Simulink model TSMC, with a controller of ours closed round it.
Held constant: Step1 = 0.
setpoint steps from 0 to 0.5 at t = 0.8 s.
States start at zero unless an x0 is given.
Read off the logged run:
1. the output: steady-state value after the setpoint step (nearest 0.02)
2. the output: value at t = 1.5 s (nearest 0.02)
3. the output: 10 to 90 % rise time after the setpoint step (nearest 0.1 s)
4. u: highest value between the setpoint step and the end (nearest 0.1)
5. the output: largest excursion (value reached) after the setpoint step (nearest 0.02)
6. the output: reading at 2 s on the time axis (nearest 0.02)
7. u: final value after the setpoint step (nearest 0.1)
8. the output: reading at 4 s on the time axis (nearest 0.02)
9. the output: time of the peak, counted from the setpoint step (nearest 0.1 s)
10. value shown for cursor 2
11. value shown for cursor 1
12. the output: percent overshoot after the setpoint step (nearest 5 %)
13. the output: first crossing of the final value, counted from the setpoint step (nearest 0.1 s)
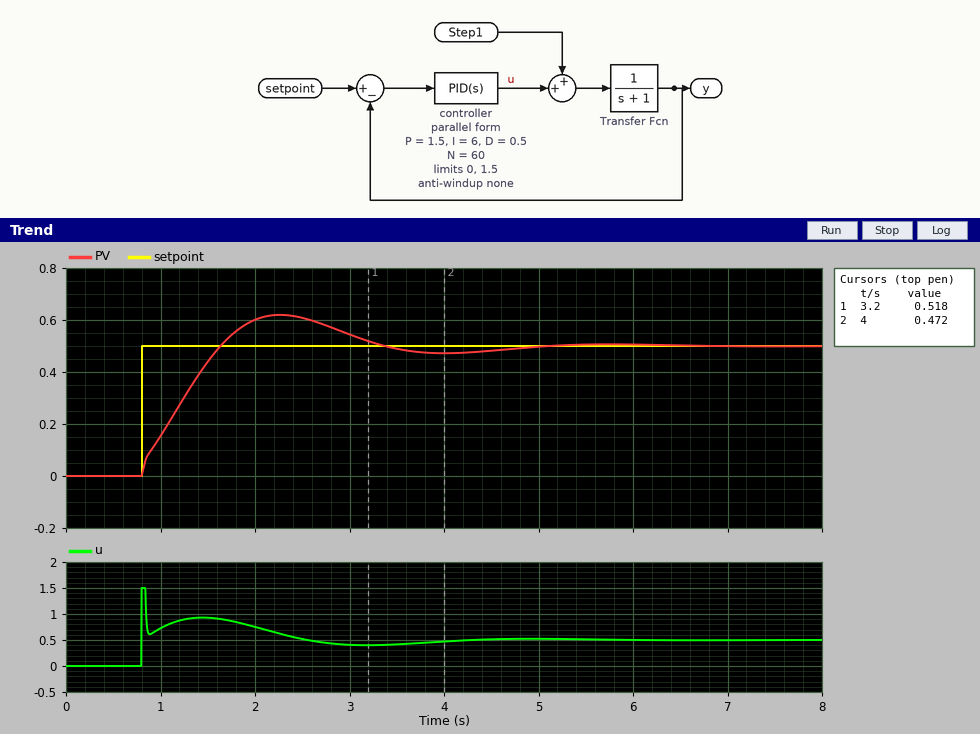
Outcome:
0.50
0.44
0.7 s
1.5
0.62
0.60
0.5
0.48
1.5 s
0.472
0.518
25 %
0.8 s
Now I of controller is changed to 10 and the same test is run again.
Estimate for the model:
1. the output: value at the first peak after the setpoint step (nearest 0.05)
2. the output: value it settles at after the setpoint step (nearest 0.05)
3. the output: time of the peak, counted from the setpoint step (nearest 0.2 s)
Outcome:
0.65
0.50
1.2 s
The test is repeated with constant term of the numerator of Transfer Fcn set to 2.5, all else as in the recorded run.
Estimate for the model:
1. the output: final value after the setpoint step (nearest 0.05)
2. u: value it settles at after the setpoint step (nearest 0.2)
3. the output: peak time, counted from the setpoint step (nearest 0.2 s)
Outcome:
0.50
0.2
1.0 s
